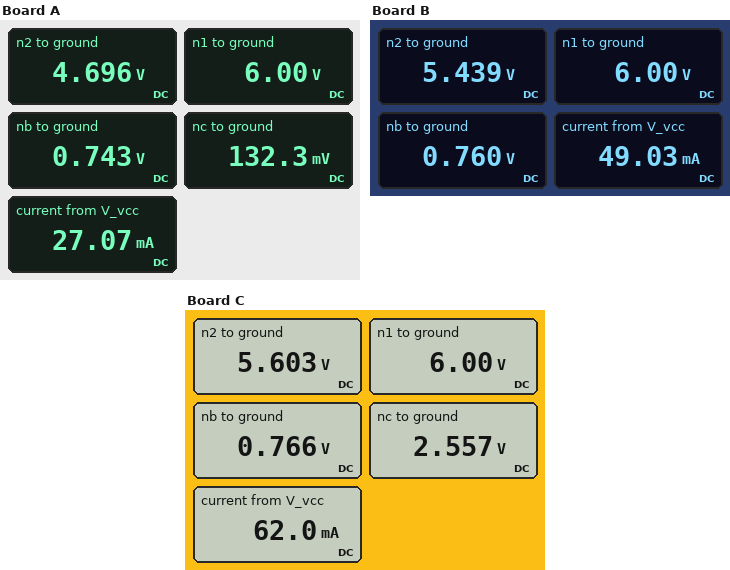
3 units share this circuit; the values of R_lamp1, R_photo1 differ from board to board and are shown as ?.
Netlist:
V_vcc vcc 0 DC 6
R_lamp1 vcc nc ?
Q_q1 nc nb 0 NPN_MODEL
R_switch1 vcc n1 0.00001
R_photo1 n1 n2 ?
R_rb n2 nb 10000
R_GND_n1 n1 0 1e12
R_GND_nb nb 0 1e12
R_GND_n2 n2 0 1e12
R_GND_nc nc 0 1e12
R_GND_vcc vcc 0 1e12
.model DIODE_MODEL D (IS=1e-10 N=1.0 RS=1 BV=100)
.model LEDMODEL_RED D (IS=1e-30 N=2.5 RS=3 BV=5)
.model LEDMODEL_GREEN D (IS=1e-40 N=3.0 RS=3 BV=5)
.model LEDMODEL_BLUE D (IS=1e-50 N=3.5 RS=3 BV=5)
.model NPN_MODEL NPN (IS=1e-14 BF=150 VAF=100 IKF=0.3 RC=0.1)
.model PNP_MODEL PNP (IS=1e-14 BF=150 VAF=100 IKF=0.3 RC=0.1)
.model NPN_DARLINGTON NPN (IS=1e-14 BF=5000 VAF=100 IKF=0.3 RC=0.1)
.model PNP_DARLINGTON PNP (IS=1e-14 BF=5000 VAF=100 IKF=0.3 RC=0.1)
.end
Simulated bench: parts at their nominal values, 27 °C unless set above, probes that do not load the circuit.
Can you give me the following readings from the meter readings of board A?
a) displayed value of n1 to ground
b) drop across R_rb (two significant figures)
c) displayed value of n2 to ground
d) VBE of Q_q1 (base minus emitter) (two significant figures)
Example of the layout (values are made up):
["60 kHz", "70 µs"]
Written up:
["6.00 V", "4.0 V", "4.696 V", "740 mV"]
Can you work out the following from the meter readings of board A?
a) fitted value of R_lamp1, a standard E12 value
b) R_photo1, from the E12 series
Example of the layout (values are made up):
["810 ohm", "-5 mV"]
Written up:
["220 Ω", "3.3 kΩ"]
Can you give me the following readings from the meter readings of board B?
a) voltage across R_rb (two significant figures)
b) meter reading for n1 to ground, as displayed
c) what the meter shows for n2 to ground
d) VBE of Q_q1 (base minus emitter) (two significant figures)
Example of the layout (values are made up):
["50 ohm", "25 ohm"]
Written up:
["4.7 V", "6.00 V", "5.439 V", "760 mV"]
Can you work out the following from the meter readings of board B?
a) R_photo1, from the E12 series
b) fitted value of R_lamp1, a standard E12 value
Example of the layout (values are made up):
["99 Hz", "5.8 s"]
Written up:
["1.2 kΩ", "120 Ω"]
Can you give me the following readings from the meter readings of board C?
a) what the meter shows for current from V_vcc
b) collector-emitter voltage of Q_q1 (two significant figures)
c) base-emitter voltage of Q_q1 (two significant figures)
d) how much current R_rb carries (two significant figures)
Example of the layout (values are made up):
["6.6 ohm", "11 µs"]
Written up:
["62.0 mA", "2.6 V", "770 mV", "480 µA"]
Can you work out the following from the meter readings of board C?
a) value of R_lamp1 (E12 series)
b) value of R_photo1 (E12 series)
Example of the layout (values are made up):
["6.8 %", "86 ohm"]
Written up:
["56 Ω", "820 Ω"]
